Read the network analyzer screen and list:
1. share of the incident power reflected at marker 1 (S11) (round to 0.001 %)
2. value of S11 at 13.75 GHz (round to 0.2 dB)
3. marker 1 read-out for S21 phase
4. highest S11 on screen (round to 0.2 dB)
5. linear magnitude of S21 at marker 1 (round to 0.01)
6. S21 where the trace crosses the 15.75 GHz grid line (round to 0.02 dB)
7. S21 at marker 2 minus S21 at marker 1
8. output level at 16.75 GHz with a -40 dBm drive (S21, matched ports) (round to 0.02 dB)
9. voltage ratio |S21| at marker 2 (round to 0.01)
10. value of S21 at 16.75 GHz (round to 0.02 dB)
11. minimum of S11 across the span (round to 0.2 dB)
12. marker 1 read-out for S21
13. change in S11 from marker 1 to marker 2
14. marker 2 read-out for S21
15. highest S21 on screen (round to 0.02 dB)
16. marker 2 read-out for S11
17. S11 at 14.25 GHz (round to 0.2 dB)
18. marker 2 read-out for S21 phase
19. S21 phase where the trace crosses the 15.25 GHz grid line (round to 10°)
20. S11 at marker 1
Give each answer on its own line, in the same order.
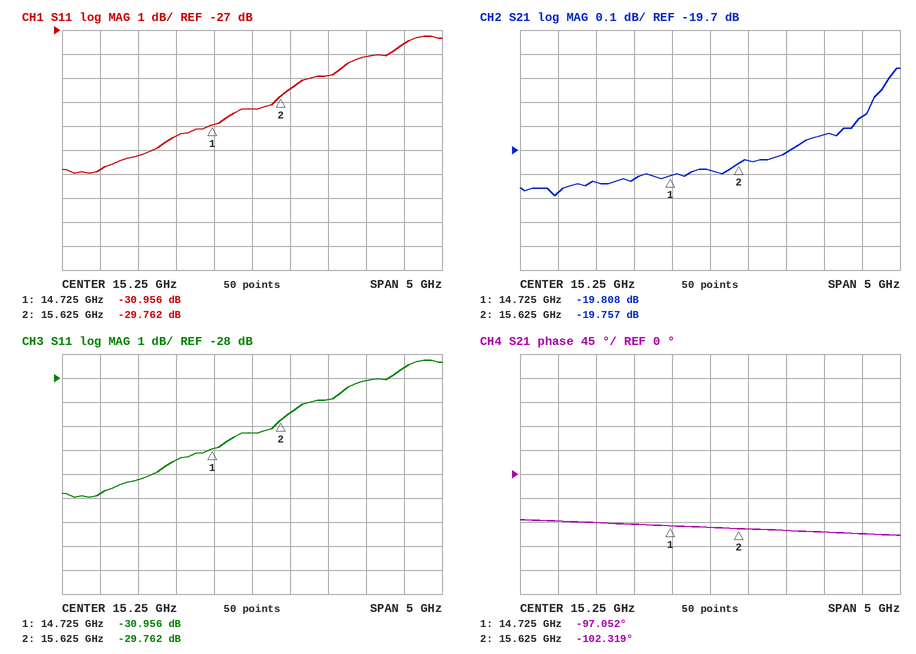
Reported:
0.080 %
-32.2 dB
-97.052°
-27.2 dB
0.10
-19.74 dB
0.051 dB
-59.64 dBm
0.10
-19.64 dB
-33.0 dB
-19.808 dB
1.194 dB
-19.757 dB
-19.36 dB
-29.762 dB
-31.4 dB
-102.319°
-100°
-30.956 dB
